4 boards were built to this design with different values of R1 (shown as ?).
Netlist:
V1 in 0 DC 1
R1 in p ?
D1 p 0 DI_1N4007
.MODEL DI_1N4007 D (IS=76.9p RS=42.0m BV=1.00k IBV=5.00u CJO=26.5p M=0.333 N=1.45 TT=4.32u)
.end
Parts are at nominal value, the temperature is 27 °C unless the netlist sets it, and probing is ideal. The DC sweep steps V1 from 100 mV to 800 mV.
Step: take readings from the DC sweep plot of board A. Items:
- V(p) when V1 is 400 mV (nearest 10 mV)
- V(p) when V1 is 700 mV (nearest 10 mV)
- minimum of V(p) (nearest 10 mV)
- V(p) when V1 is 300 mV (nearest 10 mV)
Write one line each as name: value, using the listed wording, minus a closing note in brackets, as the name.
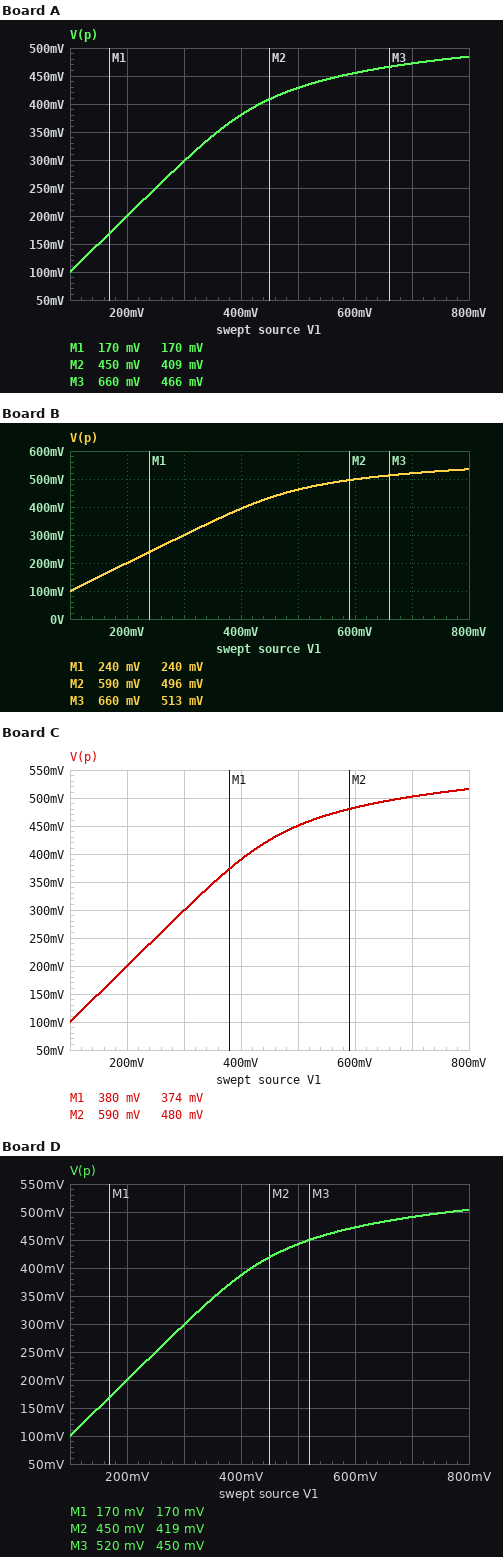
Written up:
V(p) when V1 is 400 mV: 380 mV
V(p) when V1 is 700 mV: 470 mV
minimum of V(p): 100 mV
V(p) when V1 is 300 mV: 300 mV
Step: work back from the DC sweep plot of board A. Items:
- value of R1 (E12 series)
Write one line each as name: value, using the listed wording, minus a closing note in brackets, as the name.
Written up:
value of R1: 10 kΩ
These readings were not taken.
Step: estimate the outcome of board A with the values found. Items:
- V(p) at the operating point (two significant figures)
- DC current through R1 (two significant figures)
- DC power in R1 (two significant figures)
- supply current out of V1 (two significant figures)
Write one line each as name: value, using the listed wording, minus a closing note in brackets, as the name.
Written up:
V(p) at the operating point: 500 mV
DC current through R1: 50 µA
DC power in R1: 25 µW
supply current out of V1: 50 µA
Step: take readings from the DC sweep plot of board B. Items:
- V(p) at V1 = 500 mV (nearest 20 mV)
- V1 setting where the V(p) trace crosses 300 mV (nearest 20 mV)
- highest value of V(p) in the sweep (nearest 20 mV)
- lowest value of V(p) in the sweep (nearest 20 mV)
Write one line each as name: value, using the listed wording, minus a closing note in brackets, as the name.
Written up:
V(p) at V1 = 500 mV: 460 mV
V1 setting where the V(p) trace crosses 300 mV: 300 mV
highest value of V(p) in the sweep: 540 mV
lowest value of V(p) in the sweep: 100 mV
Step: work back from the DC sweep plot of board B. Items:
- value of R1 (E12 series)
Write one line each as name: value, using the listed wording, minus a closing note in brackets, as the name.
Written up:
value of R1: 2.2 kΩ
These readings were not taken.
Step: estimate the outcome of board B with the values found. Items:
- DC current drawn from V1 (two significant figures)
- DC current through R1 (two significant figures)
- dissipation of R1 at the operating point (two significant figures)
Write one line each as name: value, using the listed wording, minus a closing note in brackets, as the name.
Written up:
DC current drawn from V1: 200 µA
DC current through R1: 200 µA
dissipation of R1 at the operating point: 90 µW
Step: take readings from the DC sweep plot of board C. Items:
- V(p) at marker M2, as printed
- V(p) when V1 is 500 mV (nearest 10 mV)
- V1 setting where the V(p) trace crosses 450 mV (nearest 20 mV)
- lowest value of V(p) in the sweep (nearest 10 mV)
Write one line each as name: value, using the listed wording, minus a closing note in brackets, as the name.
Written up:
V(p) at marker M2, as printed: 480 mV
V(p) when V1 is 500 mV: 450 mV
V1 setting where the V(p) trace crosses 450 mV: 500 mV
lowest value of V(p) in the sweep: 100 mV
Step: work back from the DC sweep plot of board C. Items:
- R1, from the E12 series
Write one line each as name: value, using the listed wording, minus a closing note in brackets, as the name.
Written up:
R1, from the E12 series: 3.9 kΩ
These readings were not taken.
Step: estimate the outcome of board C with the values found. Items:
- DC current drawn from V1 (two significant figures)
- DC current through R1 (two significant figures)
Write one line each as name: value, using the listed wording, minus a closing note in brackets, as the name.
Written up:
DC current drawn from V1: 120 µA
DC current through R1: 120 µA
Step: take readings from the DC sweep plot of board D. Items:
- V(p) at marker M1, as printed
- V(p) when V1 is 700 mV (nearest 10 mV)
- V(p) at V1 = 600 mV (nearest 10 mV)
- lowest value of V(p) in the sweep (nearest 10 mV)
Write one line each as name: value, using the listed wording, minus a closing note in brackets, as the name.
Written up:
V(p) at marker M1, as printed: 170 mV
V(p) when V1 is 700 mV: 490 mV
V(p) at V1 = 600 mV: 470 mV
lowest value of V(p) in the sweep: 100 mV
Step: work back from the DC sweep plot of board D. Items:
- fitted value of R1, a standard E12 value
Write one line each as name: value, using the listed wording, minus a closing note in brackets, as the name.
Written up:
fitted value of R1, a standard E12 value: 5.6 kΩ
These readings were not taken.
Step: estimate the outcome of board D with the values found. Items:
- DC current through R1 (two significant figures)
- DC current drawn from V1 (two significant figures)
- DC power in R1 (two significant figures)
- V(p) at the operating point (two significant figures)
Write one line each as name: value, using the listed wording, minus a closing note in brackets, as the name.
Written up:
DC current through R1: 85 µA
DC current drawn from V1: 85 µA
DC power in R1: 41 µW
V(p) at the operating point: 520 mV
